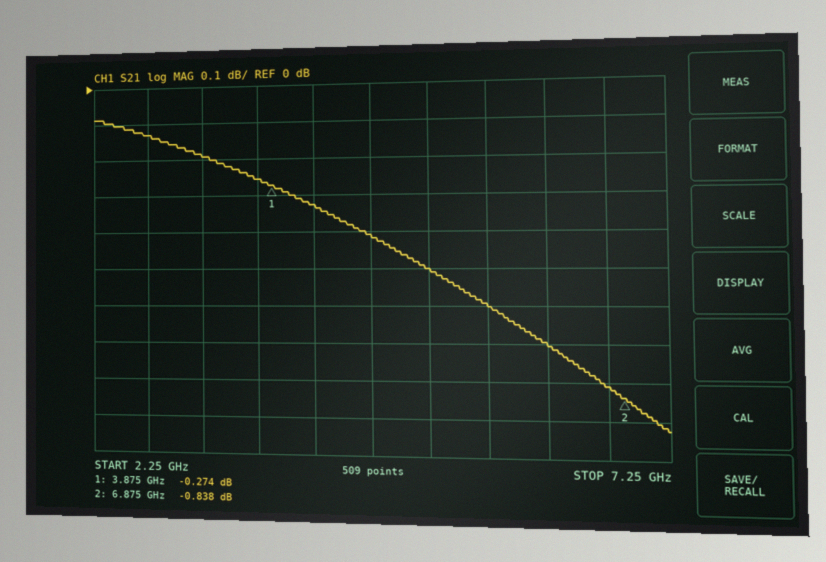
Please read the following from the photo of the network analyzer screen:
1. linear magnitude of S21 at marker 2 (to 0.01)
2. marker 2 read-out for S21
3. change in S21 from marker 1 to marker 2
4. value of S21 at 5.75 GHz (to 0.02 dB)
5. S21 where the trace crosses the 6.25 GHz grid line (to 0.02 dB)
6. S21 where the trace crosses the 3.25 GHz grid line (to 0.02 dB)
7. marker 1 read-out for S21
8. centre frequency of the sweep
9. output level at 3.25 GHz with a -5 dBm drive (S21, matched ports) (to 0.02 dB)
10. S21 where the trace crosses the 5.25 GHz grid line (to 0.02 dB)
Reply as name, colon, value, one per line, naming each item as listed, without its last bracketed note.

linear magnitude of S21 at marker 2: 0.91
marker 2 read-out for S21: -0.838 dB
change in S21 from marker 1 to marker 2: -0.564 dB
value of S21 at 5.75 GHz: -0.60 dB
S21 where the trace crosses the 6.25 GHz grid line: -0.70 dB
S21 where the trace crosses the 3.25 GHz grid line: -0.20 dB
marker 1 read-out for S21: -0.274 dB
centre frequency of the sweep: 4.75 GHz
output level at 3.25 GHz with a -5 dBm drive (S21, matched ports): -5.20 dBm
S21 where the trace crosses the 5.25 GHz grid line: -0.50 dB
